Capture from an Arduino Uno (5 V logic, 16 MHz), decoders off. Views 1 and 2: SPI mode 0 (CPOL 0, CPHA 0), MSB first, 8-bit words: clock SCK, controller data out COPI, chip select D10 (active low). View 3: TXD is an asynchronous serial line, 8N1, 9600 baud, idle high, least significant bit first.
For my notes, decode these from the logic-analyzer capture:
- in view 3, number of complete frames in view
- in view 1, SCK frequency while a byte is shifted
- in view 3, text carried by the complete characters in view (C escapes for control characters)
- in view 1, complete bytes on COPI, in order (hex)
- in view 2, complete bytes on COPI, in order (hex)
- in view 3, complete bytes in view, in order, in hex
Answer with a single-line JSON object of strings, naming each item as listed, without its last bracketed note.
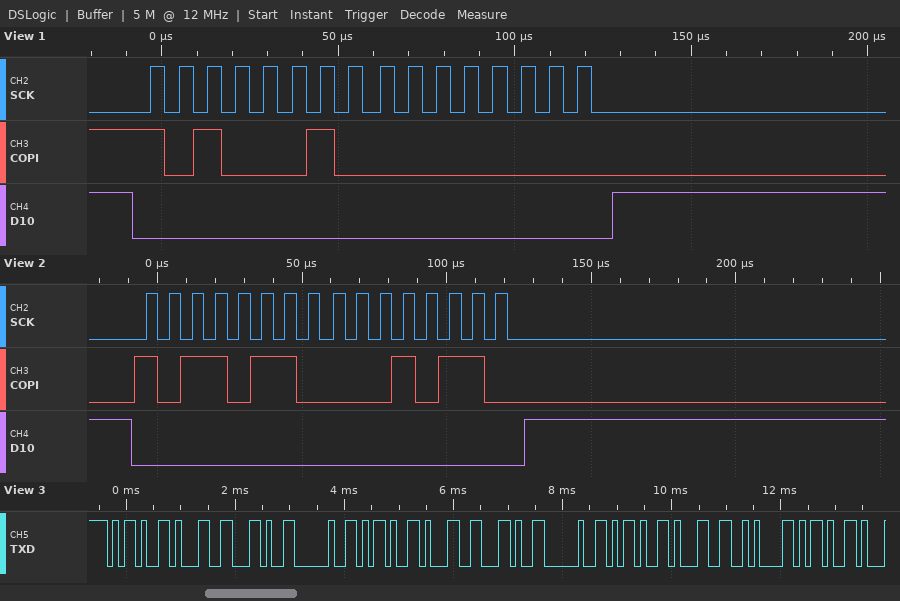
{"in view 3, number of complete frames in view": "12", "in view 1, SCK frequency while a byte is shifted": "125 kHz", "in view 3, text carried by the complete characters in view": "\"-1, -1, -1\\n-\"", "in view 1, complete bytes on COPI, in order": "0xA2 0x00", "in view 2, complete bytes on COPI, in order": "B6 16", "in view 3, complete bytes in view, in order, in hex": "0x2D 0x31 0x2C 0x20 0x2D 0x31 0x2C 0x20 0x2D 0x31 0x0A 0x2D"}
